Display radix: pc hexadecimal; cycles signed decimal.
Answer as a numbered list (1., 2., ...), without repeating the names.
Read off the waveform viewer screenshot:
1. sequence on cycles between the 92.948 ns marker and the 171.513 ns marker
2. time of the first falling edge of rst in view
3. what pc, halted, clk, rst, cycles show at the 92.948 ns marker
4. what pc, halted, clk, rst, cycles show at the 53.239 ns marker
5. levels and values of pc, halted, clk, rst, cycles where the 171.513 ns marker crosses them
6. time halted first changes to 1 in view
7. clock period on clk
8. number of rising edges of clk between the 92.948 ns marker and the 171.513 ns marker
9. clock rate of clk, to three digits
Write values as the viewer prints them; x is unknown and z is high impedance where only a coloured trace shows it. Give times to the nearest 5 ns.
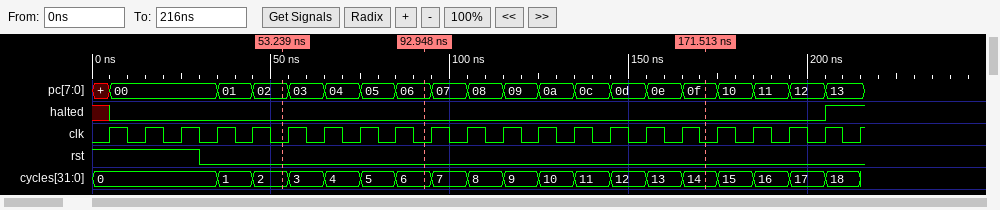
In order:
1. 6, 7, 8, 9, 10, 11, 12, 13, 14
2. 30 ns
3. pc=06, halted=0, clk=0, rst=0, cycles=6
4. pc=02, halted=0, clk=0, rst=0, cycles=2
5. pc=0f, halted=0, clk=0, rst=0, cycles=14
6. 205 ns
7. 10 ns
8. 8
9. 100 MHz
